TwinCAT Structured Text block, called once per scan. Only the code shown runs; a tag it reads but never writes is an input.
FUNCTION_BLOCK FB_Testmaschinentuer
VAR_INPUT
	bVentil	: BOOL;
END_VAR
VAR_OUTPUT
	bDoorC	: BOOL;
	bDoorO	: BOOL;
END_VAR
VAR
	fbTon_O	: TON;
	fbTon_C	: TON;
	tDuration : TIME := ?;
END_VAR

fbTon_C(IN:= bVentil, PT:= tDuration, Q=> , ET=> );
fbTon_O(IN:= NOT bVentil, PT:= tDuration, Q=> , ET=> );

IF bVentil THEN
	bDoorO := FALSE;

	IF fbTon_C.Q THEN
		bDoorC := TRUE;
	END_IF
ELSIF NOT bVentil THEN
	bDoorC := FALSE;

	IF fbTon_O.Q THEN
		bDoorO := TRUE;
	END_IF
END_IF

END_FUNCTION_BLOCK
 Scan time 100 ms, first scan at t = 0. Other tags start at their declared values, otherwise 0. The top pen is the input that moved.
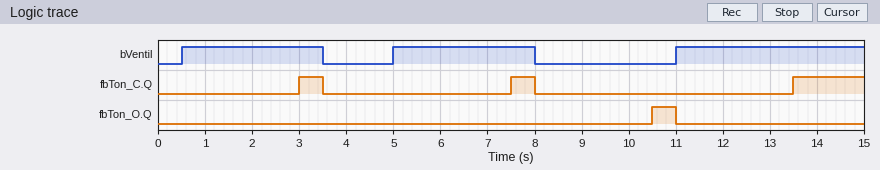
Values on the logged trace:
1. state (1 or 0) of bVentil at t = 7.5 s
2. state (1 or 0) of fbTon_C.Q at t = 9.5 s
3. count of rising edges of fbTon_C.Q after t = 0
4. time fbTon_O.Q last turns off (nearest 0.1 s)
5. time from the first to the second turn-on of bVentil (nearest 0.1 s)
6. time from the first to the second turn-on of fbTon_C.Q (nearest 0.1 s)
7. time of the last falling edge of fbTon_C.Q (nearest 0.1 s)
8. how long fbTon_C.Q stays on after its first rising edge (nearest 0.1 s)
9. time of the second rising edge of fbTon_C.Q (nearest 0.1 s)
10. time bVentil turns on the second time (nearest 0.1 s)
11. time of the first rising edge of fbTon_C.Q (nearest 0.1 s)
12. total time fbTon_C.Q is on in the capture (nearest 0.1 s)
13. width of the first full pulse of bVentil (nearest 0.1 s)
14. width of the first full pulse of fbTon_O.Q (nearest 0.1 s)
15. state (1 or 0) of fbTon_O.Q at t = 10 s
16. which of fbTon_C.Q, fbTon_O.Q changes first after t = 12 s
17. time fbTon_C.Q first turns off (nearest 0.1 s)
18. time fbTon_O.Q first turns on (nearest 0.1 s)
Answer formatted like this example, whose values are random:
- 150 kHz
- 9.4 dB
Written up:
- 1
- 0
- 3
- 11.0 s
- 4.5 s
- 4.5 s
- 8.0 s
- 0.5 s
- 7.5 s
- 5.0 s
- 3.0 s
- 2.5 s
- 3.0 s
- 0.5 s
- 0
- fbTon_C.Q
- 3.5 s
- 10.5 s
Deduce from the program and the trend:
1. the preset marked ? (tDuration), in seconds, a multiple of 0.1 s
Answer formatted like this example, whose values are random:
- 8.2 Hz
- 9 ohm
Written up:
- 2.5 s
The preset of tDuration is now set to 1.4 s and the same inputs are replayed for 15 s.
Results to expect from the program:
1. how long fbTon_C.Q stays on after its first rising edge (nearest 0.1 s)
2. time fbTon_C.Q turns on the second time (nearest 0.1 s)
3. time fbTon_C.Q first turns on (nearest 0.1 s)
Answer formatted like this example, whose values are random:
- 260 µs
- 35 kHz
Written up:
- 1.6 s
- 6.4 s
- 1.9 s
